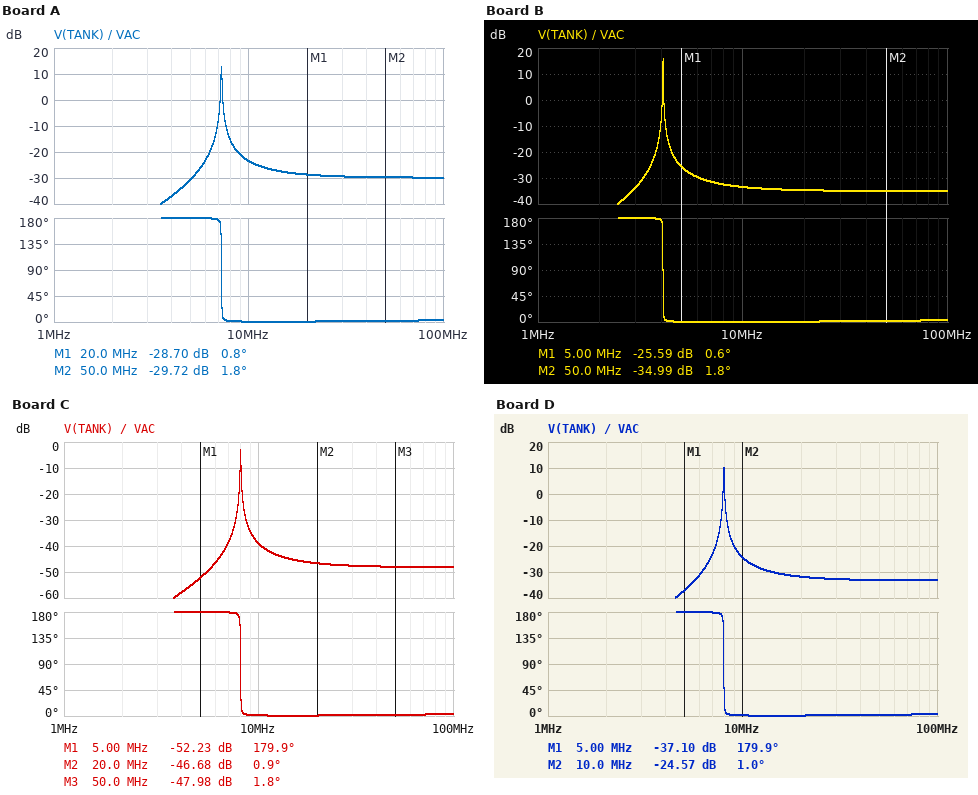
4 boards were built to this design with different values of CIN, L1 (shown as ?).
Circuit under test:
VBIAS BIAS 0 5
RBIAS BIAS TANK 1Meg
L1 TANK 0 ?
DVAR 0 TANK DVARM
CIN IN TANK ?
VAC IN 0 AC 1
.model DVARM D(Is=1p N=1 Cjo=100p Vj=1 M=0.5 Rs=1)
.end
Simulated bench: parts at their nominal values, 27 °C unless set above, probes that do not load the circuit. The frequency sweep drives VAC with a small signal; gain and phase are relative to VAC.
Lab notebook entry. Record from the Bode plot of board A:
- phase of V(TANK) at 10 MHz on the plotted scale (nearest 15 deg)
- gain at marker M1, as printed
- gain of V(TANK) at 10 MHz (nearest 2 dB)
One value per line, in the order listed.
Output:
0 deg
-28.70 dB
-24 dB
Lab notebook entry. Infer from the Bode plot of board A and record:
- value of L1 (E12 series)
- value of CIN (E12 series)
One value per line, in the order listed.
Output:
4.7 µH
3.3 pF
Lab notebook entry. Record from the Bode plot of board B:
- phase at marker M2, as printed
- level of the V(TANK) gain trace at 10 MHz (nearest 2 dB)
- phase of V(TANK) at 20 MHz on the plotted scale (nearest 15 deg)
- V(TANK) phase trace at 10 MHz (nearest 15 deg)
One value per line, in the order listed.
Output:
1.8 deg
-34 dB
0 deg
0 deg
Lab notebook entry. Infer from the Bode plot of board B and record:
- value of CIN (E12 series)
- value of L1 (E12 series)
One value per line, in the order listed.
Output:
1.8 pF
15 µH
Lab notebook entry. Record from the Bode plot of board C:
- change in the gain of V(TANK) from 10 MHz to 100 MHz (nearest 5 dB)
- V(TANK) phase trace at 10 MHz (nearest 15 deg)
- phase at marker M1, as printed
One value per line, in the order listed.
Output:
-10 dB
0 deg
179.9 deg
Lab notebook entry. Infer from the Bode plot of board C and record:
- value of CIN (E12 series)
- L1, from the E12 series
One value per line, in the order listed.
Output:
390 fF
3.9 µH
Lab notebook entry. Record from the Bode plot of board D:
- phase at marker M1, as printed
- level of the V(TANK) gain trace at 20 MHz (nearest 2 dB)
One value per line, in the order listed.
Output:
179.9 deg
-32 dB
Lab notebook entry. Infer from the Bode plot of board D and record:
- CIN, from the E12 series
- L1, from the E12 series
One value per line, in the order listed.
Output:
2.2 pF
3.9 µH
